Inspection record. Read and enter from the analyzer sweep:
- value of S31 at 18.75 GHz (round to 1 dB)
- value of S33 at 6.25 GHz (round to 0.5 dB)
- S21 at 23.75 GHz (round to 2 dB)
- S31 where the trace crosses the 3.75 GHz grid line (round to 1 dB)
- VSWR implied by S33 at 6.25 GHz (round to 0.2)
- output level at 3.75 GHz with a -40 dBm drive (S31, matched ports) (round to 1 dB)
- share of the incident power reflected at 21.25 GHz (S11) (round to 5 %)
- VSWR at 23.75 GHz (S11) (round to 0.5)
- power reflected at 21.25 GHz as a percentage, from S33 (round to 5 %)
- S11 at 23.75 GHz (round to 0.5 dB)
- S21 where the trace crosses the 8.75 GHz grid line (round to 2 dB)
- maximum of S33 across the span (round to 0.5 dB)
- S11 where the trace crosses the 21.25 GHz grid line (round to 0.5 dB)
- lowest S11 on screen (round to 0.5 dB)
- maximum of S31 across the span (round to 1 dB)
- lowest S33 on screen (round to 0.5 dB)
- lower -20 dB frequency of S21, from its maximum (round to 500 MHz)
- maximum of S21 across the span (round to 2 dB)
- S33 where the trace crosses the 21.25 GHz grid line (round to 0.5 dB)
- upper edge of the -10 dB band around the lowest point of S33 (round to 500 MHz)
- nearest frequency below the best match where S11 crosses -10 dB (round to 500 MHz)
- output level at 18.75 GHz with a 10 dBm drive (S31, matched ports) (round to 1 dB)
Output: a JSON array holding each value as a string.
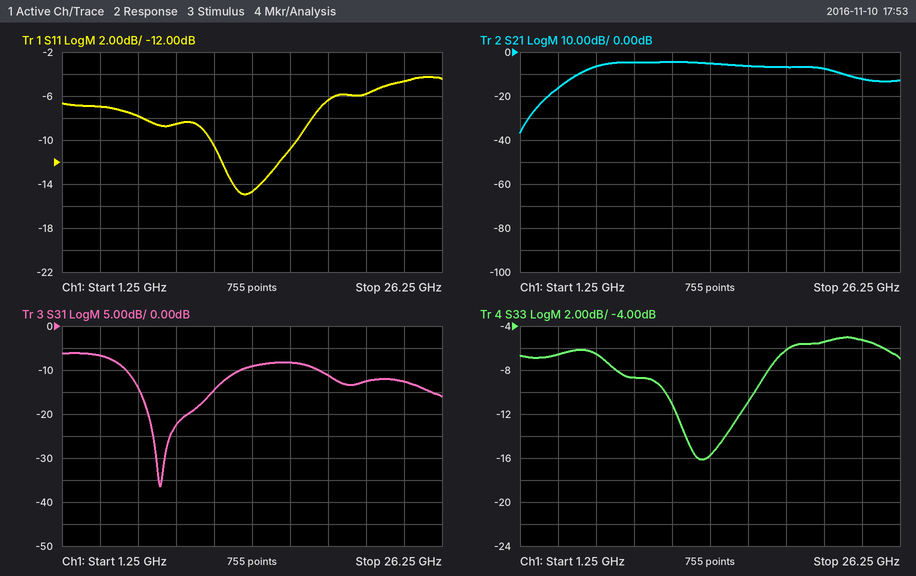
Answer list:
["-11 dB", "-6.5 dB", "-12 dB", "-7 dB", "2.8", "-47 dBm", "25 %", "4.0", "30 %", "-4.5 dB", "-4 dB", "-5.0 dB", "-6.0 dB", "-15.0 dB", "-6 dB", "-16.0 dB", "2.5 GHz", "-4 dB", "-5.5 dB", "16.5 GHz", "11.0 GHz", "-1 dBm"]
